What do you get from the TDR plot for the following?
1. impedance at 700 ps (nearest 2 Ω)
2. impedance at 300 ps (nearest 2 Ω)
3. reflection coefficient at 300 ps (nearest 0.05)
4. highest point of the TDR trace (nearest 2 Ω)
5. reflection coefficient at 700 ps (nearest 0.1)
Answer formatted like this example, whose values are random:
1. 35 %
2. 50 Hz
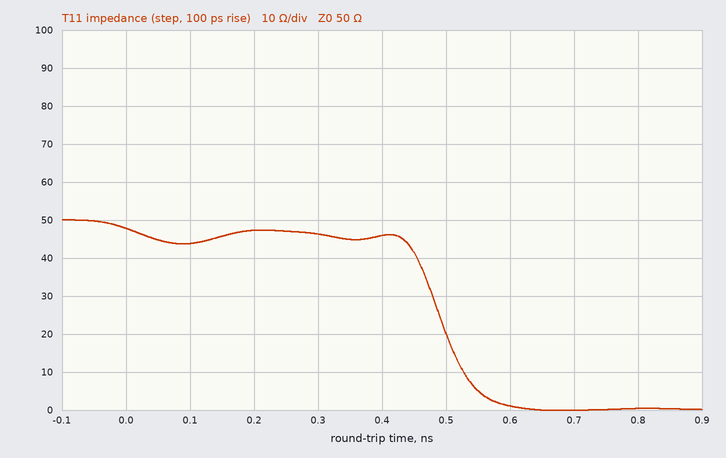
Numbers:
1. 0 Ω
2. 46 Ω
3. -0.05
4. 50 Ω
5. -1.0
